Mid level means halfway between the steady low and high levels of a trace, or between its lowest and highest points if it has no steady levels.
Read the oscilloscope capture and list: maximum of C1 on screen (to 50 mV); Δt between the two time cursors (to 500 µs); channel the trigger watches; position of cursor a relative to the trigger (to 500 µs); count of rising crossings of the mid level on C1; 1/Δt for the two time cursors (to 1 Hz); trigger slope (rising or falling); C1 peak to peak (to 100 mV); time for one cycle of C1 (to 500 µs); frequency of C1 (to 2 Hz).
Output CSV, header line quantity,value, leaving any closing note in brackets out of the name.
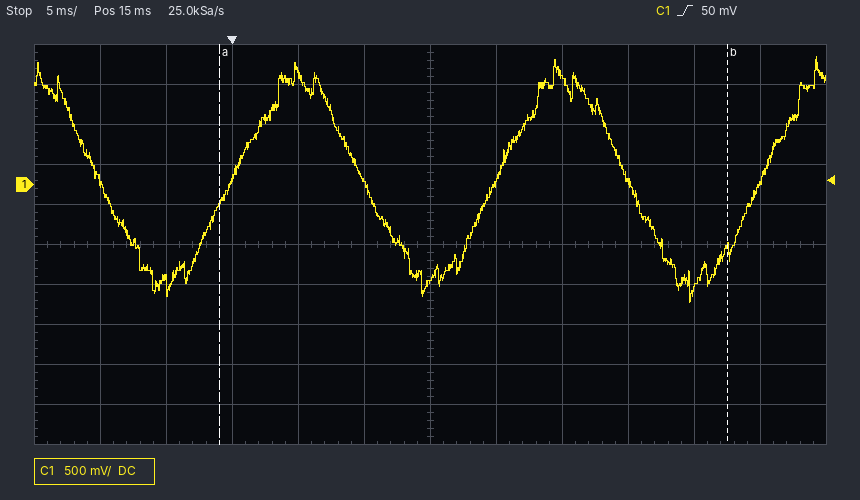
quantity,value
maximum of C1 on screen,1.60 V
Δt between the two time cursors,38.5 ms
channel the trigger watches,C1
position of cursor a relative to the trigger,-1.0 ms
count of rising crossings of the mid level on C1,3
1/Δt for the two time cursors,26 Hz
trigger slope,rising
C1 peak to peak,3.10 V
time for one cycle of C1,20.0 ms
frequency of C1,50 Hz
